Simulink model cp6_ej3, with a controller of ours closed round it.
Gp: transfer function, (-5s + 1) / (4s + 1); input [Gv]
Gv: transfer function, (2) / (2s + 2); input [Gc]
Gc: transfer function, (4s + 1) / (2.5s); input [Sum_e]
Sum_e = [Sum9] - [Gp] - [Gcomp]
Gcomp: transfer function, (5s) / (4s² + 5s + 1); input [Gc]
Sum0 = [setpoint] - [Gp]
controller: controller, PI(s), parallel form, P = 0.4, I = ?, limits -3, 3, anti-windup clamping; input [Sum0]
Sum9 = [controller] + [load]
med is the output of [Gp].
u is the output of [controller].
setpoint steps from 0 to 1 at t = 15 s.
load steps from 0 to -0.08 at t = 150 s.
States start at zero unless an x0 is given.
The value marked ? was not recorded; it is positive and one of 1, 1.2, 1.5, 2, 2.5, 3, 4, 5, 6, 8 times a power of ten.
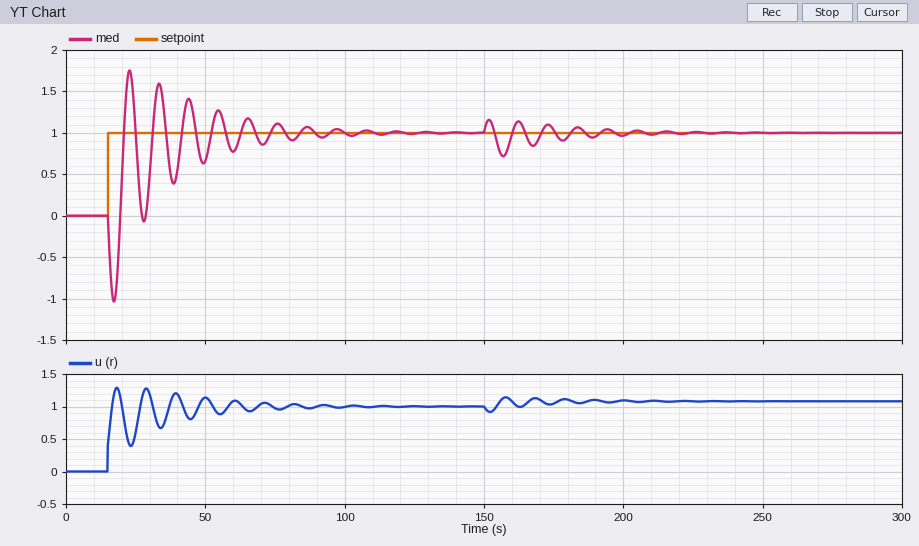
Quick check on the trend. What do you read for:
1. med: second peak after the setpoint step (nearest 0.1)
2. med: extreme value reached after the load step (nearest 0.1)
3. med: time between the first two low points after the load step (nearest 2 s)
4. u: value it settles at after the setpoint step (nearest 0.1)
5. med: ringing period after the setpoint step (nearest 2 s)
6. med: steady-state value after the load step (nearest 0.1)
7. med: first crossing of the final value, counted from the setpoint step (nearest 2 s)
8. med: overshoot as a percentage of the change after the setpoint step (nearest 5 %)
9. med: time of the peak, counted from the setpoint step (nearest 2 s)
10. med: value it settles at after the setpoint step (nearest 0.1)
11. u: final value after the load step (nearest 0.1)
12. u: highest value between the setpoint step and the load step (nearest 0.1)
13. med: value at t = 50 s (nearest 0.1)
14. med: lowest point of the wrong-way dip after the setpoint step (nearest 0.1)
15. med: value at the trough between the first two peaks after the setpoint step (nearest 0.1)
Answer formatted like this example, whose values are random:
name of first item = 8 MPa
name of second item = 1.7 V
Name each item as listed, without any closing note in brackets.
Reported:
med: second peak after the setpoint step = 1.6
med: extreme value reached after the load step = 0.7
med: time between the first two low points after the load step = 10 s
u: value it settles at after the setpoint step = 1.0
med: ringing period after the setpoint step = 10 s
med: steady-state value after the load step = 1.0
med: first crossing of the final value, counted from the setpoint step = 6 s
med: overshoot as a percentage of the change after the setpoint step = 75 %
med: time of the peak, counted from the setpoint step = 8 s
med: value it settles at after the setpoint step = 1.0
u: final value after the load step = 1.1
u: highest value between the setpoint step and the load step = 1.3
med: value at t = 50 s = 0.7
med: lowest point of the wrong-way dip after the setpoint step = -1.0
med: value at the trough between the first two peaks after the setpoint step = -0.1
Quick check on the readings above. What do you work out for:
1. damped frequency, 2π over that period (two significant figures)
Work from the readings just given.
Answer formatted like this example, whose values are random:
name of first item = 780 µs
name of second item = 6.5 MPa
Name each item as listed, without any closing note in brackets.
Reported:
damped frequency, 2π over that period = 0.63 rad/s
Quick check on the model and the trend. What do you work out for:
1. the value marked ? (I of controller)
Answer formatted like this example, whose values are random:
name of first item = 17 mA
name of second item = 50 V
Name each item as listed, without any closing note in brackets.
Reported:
the value marked ? = 0.1
